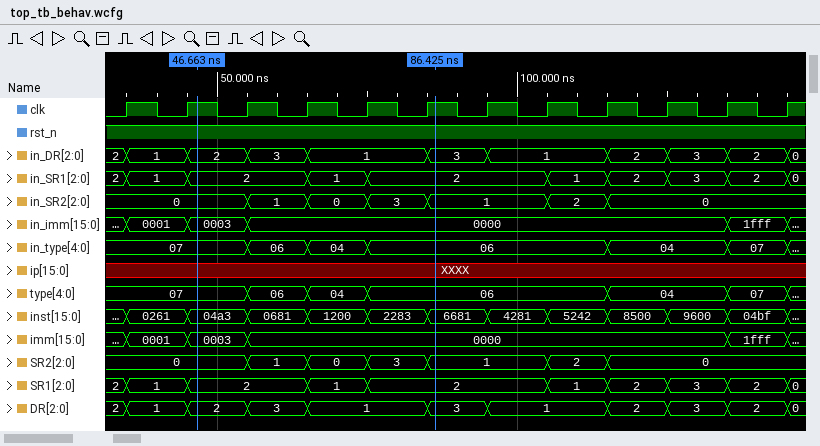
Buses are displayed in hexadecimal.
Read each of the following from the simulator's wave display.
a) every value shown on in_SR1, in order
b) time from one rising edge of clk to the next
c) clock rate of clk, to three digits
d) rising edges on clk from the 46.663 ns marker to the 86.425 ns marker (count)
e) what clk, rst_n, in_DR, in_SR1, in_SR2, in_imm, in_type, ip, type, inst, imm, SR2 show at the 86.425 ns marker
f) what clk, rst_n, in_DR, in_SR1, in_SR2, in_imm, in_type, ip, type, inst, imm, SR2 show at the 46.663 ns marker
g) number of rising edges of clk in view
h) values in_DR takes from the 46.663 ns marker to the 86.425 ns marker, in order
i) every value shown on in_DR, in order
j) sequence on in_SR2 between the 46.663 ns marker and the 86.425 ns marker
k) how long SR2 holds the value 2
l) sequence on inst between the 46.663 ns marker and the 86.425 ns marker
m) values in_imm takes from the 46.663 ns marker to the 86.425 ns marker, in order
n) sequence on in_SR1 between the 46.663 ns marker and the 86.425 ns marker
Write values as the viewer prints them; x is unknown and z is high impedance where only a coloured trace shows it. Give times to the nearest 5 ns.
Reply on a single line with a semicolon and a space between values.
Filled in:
2, 1, 2, 1, 2, 1, 2, 3, 2, 0; 10 ns; 100 MHz; 4; clk=1, rst_n=1, in_DR=3, in_SR1=2, in_SR2=1, in_imm=0000, in_type=06, ip=XXXX, type=06, inst=6681, imm=0000, SR2=1; clk=1, rst_n=1, in_DR=2, in_SR1=2, in_SR2=0, in_imm=0003, in_type=07, ip=XXXX, type=07, inst=04a3, imm=0003, SR2=0; 12; 2, 3, 1, 3; 2, 1, 2, 3, 1, 3, 1, 2, 3, 2, 0; 0, 1, 0, 3, 1; 10 ns; 04a3, 0681, 1200, 2283, 6681; 0003, 0000; 2, 1, 2
